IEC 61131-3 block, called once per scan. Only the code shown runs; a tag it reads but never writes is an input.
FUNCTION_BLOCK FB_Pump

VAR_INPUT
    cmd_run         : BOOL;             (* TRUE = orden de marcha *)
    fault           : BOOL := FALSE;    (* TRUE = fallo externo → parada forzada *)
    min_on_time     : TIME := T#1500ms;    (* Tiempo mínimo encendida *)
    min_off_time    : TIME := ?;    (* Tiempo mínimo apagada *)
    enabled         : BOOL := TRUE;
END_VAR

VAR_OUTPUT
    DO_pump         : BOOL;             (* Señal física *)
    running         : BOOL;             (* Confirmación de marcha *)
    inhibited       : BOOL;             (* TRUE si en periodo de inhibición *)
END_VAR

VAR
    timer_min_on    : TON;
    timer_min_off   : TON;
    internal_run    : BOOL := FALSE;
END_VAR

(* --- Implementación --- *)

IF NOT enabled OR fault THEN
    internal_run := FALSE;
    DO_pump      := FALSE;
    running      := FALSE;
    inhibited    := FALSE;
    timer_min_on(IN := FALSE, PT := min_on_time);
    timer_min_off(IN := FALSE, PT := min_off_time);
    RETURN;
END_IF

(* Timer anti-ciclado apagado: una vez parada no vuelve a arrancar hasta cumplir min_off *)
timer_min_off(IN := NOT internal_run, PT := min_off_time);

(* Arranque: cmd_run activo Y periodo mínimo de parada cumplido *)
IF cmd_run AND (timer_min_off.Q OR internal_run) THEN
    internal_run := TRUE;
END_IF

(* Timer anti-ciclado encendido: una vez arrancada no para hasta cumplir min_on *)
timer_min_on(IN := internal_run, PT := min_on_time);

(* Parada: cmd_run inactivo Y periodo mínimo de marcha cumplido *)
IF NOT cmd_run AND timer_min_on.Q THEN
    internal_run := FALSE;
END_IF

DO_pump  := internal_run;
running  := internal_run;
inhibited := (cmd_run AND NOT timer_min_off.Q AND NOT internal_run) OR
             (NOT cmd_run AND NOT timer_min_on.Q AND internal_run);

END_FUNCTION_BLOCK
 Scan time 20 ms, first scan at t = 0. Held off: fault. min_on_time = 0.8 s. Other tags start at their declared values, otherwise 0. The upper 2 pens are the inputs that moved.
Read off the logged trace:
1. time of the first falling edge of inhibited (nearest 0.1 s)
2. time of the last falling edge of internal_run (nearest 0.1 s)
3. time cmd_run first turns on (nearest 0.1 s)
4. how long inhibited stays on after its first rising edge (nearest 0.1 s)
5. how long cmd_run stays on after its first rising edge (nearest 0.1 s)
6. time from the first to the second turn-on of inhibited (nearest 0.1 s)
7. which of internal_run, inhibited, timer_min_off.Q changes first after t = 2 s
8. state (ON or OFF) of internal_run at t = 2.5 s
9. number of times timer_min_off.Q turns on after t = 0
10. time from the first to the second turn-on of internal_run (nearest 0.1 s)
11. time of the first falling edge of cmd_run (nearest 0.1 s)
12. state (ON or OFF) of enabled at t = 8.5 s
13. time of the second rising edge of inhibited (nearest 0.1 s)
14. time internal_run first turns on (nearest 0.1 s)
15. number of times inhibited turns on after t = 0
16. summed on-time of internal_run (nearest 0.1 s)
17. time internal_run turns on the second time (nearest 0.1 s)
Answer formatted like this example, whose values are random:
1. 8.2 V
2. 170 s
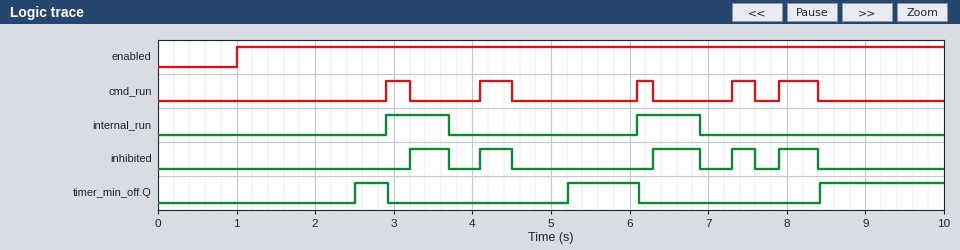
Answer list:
1. 3.7 s
2. 6.9 s
3. 2.9 s
4. 0.5 s
5. 0.3 s
6. 0.9 s
7. timer_min_off.Q
8. OFF
9. 3
10. 3.2 s
11. 3.2 s
12. ON
13. 4.1 s
14. 2.9 s
15. 5
16. 1.6 s
17. 6.1 s
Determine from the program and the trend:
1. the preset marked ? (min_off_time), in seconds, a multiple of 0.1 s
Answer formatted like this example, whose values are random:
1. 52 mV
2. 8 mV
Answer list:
1. 1.5 s
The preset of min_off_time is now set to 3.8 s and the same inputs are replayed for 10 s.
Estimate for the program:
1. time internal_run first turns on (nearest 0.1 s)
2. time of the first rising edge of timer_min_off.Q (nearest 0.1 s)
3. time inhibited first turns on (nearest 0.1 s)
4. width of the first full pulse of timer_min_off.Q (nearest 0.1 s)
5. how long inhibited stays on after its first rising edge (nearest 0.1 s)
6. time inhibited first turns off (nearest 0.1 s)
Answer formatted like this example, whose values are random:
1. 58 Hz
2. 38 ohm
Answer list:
1. 6.1 s
2. 4.8 s
3. 2.9 s
4. 1.3 s
5. 0.3 s
6. 3.2 s
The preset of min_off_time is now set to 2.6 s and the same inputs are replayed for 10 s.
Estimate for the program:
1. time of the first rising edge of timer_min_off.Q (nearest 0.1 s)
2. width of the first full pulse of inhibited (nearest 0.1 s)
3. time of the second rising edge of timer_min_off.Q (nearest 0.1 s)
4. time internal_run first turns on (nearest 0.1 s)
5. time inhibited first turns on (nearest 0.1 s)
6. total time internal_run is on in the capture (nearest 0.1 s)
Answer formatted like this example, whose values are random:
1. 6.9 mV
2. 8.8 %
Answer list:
1. 3.6 s
2. 0.3 s
3. 7.5 s
4. 4.1 s
5. 2.9 s
6. 1.7 s
